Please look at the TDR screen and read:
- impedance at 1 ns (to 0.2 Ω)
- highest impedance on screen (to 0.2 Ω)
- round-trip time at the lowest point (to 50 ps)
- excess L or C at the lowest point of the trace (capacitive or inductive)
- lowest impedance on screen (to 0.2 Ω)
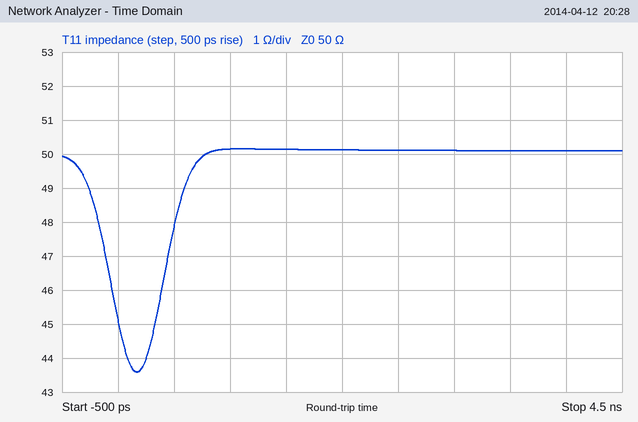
50.2 Ω
50.2 Ω
150 ps
capacitive
43.6 Ω
